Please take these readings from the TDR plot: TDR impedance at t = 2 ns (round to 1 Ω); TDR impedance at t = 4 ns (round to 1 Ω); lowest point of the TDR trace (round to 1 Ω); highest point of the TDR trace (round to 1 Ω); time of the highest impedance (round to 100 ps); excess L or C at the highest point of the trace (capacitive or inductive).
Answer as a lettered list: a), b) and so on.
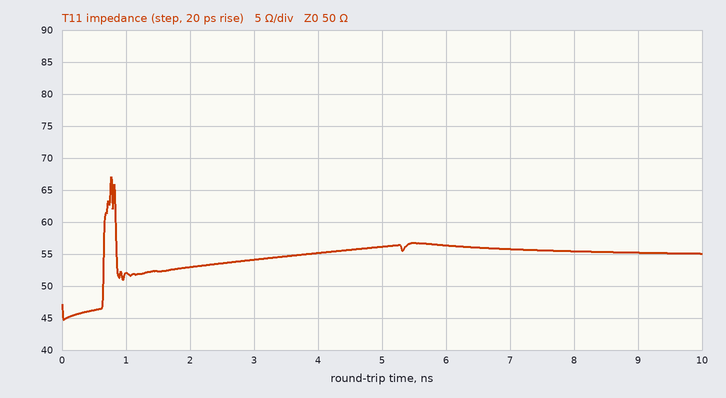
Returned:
a) 53 Ω
b) 55 Ω
c) 45 Ω
d) 67 Ω
e) 800 ps
f) inductive
